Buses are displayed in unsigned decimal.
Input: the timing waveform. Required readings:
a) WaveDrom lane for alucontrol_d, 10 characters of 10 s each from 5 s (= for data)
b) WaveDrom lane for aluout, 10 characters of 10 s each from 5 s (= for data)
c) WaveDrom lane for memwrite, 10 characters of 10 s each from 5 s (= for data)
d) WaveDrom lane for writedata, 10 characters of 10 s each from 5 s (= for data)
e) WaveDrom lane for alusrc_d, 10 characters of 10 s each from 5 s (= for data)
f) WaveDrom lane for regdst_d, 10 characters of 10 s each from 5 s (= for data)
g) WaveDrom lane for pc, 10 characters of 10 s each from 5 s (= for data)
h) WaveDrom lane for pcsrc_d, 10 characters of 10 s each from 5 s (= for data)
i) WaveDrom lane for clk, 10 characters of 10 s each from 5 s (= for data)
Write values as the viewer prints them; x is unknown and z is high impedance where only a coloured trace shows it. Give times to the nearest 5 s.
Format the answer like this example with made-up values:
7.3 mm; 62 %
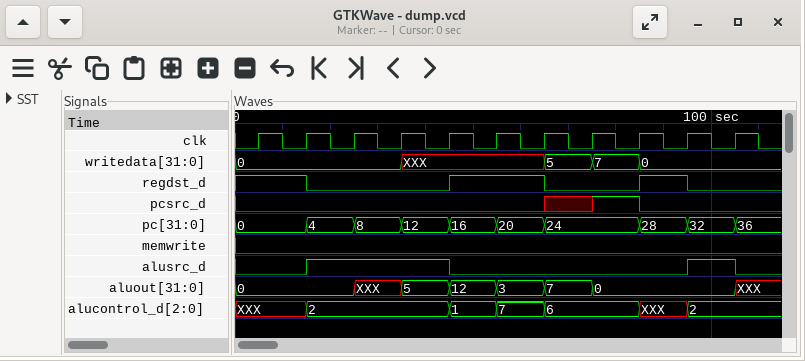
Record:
{name: 'alucontrol_d', wave: 'x=..===.x=', data: '2 1 7 6 2'}; {name: 'aluout', wave: '=.x=====..', data: '0 5 12 3 7 0'}; {name: 'memwrite', wave: '0.........'}; {name: 'writedata', wave: '=..x..===.', data: '0 5 7 0'}; {name: 'alusrc_d', wave: '01..0....1'}; {name: 'regdst_d', wave: '10..1.0.10'}; {name: 'pc', wave: '=======.==', data: '0 4 8 12 16 20 24 28 32'}; {name: 'pcsrc_d', wave: '0.....x10.'}; {name: 'clk', wave: 'p.........'}
